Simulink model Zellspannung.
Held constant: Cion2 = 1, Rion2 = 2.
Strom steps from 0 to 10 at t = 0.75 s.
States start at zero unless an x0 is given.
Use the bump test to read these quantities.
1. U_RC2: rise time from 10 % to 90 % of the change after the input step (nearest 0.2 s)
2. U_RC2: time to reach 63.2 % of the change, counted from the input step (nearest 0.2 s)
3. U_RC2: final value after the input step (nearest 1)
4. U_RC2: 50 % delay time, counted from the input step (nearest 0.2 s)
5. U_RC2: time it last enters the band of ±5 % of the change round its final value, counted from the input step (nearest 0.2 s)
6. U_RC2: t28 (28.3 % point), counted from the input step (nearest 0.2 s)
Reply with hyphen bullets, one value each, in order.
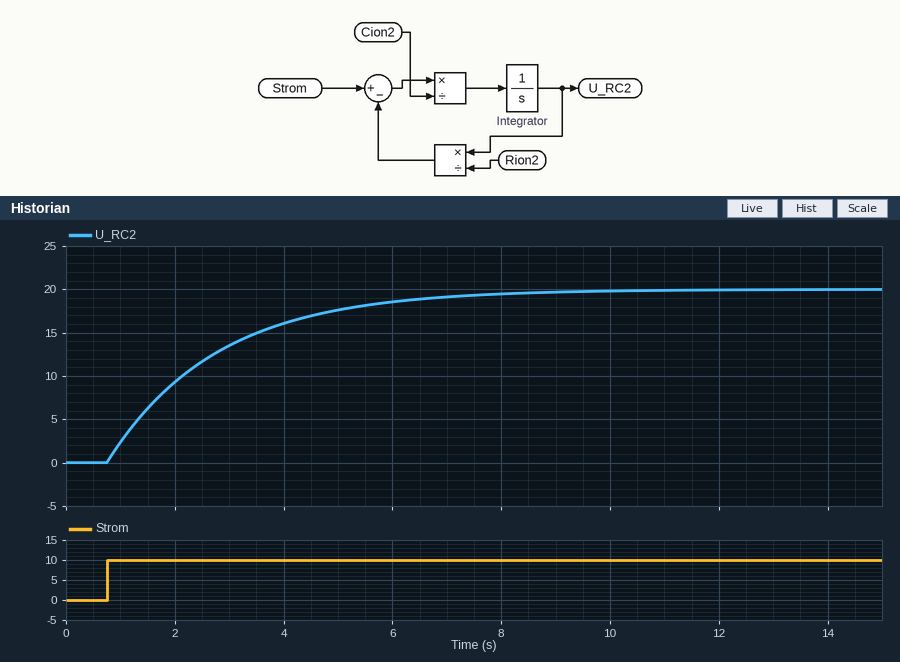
- 4.4 s
- 2.0 s
- 20
- 1.4 s
- 6.0 s
- 0.6 s
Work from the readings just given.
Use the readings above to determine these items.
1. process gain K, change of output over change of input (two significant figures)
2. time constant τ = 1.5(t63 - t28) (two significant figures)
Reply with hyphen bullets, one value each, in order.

- 2.0
- 2.1 s
